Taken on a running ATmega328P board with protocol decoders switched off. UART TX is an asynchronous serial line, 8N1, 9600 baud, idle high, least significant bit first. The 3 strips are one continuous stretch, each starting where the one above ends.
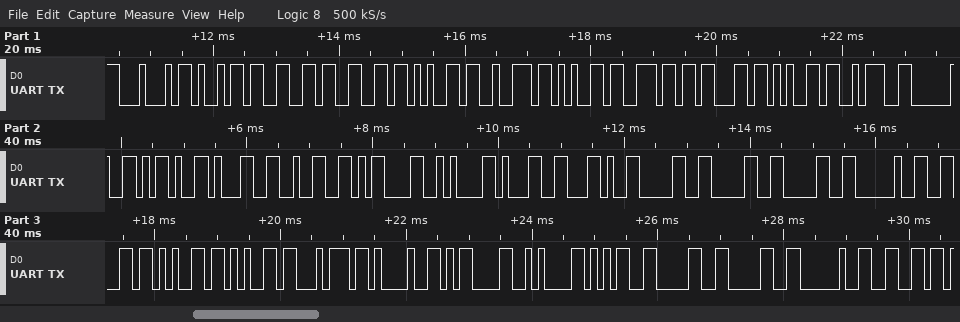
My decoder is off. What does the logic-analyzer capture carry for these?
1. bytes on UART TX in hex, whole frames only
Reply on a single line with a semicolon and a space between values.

0x44 0x69 0x66 0x66 0x65 0x72 0x65 0x6E 0x63 0x65 0x3A 0x20 0x2D 0x31 0x32 0x0D 0x0A 0x31 0x2C 0x30 0x30 0x30 0x20 0x66 0x65 0x65 0x74 0x21 0x0D 0x0A 0x35 0x30 0x30 0x20 0x66
